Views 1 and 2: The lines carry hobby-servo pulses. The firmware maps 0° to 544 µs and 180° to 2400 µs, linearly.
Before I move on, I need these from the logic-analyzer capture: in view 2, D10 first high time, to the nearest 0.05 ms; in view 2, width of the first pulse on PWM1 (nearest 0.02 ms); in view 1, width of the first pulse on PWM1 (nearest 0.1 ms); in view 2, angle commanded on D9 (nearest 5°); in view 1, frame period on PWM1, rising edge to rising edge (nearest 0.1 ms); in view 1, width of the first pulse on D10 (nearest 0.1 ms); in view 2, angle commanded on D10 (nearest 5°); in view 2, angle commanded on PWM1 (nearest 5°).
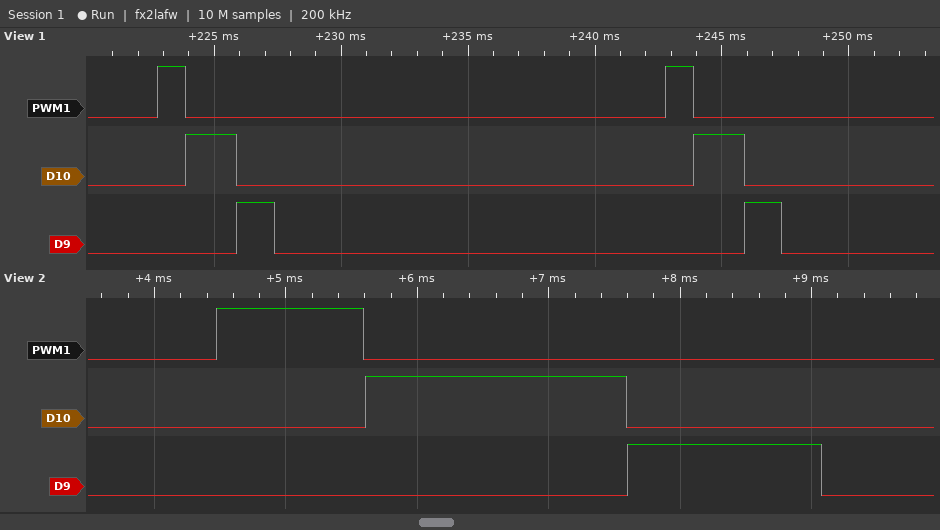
2.00 ms
1.12 ms
1.1 ms
90°
20.0 ms
2.0 ms
140°
55°
